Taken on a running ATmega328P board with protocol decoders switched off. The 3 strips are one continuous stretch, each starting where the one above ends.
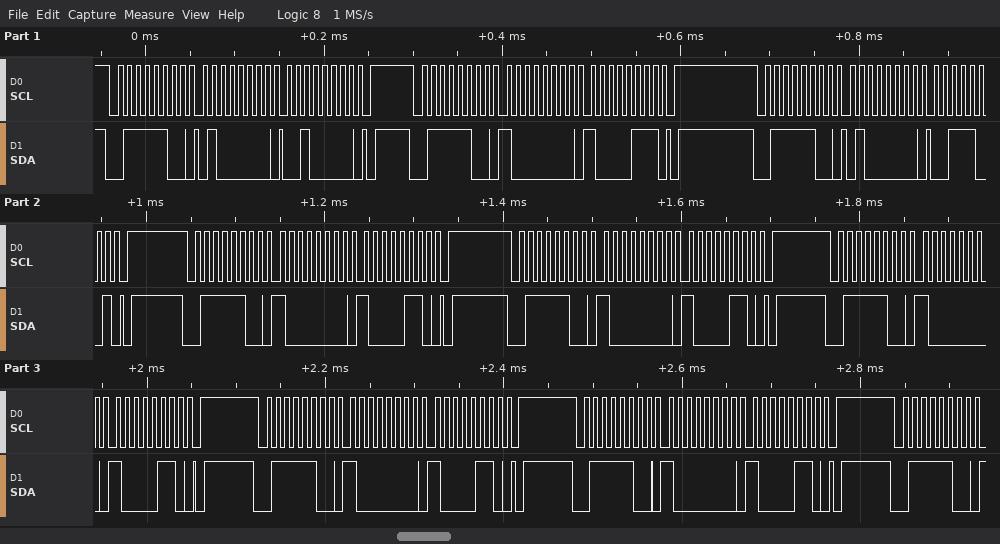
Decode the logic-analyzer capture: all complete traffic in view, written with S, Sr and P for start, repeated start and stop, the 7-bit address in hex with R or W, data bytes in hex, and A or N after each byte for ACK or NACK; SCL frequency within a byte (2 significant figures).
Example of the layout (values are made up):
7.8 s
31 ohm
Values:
S 3EW A 40 A 20 A P S 3EW A 80 A 87 A P S 3EW A 40 A 39 A P S 3EW A 80 A 86 A P S 3EW A 80 A 86 A P S 3EW A 80 A 86 A P S 3EW A 80 A 86 A P S 3EW A 80 A 86 A P S 3EW A
100 kHz
